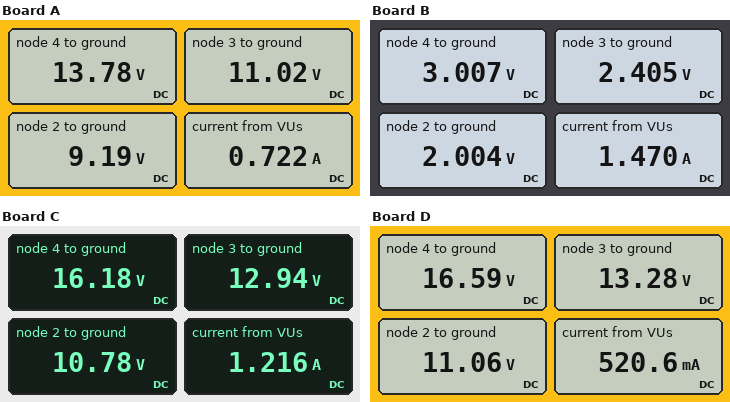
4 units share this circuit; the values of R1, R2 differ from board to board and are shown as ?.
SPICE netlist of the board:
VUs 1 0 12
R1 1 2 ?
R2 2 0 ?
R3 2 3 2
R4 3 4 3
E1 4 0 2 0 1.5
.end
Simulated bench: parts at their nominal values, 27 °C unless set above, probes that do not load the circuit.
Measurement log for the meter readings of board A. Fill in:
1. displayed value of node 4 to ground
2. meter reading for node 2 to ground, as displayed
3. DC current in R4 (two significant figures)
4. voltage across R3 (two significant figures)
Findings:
13.78 V
9.19 V
920 mA
1.8 V
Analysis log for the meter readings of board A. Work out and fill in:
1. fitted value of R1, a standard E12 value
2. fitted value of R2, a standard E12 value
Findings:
3.9 Ω
5.6 Ω
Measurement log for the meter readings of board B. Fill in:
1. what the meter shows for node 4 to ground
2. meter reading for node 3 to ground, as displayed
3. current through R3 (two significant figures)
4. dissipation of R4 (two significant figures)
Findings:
3.007 V
2.405 V
200 mA
120 mW
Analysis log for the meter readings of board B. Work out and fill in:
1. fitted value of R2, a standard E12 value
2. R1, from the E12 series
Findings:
1.2 Ω
6.8 Ω
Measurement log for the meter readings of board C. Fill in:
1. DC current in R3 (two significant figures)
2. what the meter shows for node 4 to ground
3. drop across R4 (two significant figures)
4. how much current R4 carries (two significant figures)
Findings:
1.1 A
16.18 V
3.2 V
1.1 A
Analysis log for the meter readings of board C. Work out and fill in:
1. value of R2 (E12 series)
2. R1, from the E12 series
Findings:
4.7 Ω
1 Ω
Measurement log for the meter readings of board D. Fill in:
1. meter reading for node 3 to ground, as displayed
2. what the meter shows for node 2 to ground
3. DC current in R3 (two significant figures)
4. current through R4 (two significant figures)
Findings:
13.28 V
11.06 V
1.1 A
1.1 A
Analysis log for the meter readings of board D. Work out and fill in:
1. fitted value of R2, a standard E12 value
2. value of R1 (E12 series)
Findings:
6.8 Ω
1.8 Ω
